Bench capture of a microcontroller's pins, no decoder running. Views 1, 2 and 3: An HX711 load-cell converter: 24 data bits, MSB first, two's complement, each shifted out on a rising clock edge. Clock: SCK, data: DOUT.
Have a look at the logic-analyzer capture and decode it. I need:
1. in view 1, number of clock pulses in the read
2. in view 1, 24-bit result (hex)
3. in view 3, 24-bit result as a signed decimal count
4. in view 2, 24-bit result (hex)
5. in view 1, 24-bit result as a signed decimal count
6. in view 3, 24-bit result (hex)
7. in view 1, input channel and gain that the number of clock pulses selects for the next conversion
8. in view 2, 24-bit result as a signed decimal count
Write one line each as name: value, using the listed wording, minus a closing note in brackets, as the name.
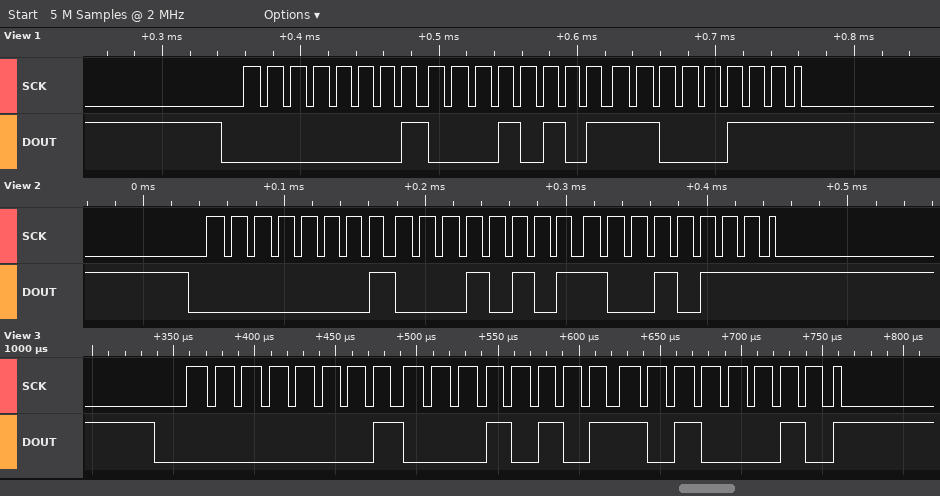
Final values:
in view 1, number of clock pulses in the read: 25
in view 1, 24-bit result: 0x0115C7
in view 3, 24-bit result as a signed decimal count: 71074
in view 2, 24-bit result: 0x011597
in view 1, 24-bit result as a signed decimal count: 71111
in view 3, 24-bit result: 0x0115A2
in view 1, input channel and gain that the number of clock pulses selects for the next conversion: channel A, gain 128
in view 2, 24-bit result as a signed decimal count: 71063
